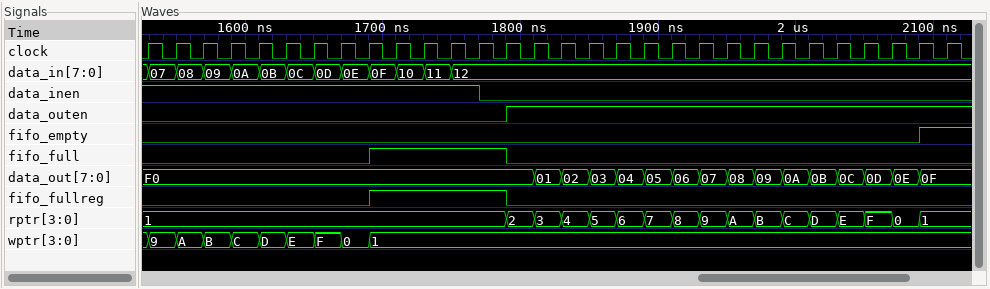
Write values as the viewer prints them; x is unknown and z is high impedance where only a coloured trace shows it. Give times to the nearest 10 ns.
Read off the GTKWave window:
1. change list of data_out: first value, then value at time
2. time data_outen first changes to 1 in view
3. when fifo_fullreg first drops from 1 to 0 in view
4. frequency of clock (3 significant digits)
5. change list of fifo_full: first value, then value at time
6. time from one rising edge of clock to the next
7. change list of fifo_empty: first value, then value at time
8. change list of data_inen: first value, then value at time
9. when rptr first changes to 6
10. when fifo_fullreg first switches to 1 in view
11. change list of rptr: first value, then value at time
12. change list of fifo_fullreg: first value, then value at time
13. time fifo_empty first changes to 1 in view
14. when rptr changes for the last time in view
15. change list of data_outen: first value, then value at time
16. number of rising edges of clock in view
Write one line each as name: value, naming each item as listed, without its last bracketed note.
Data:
change list of data_out: first value, then value at time: F0, 01 at 1810 ns, 02 at 1830 ns, 03 at 1850 ns, 04 at 1870 ns, 05 at 1890 ns, 06 at 1910 ns, 07 at 1930 ns, 08 at 1950 ns, 09 at 1970 ns, 0A at 1990 ns, 0B at 2010 ns, 0C at 2030 ns, 0D at 2050 ns, 0E at 2070 ns, 0F at 2090 ns
time data_outen first changes to 1 in view: 1790 ns
when fifo_fullreg first drops from 1 to 0 in view: 1790 ns
frequency of clock: 50.0 MHz
change list of fifo_full: first value, then value at time: 0, 1 at 1690 ns, 0 at 1790 ns
time from one rising edge of clock to the next: 20 ns
change list of fifo_empty: first value, then value at time: 0, 1 at 2090 ns
change list of data_inen: first value, then value at time: 1, 0 at 1770 ns
when rptr first changes to 6: 1870 ns
when fifo_fullreg first switches to 1 in view: 1690 ns
change list of rptr: first value, then value at time: 1, 2 at 1790 ns, 3 at 1810 ns, 4 at 1830 ns, 5 at 1850 ns, 6 at 1870 ns, 7 at 1890 ns, 8 at 1910 ns, 9 at 1930 ns, A at 1950 ns, B at 1970 ns, C at 1990 ns, D at 2010 ns, E at 2030 ns, F at 2050 ns, 0 at 2070 ns, 1 at 2090 ns
change list of fifo_fullreg: first value, then value at time: 0, 1 at 1690 ns, 0 at 1790 ns
time fifo_empty first changes to 1 in view: 2090 ns
when rptr changes for the last time in view: 2090 ns
change list of data_outen: first value, then value at time: 0, 1 at 1790 ns
number of rising edges of clock in view: 30
